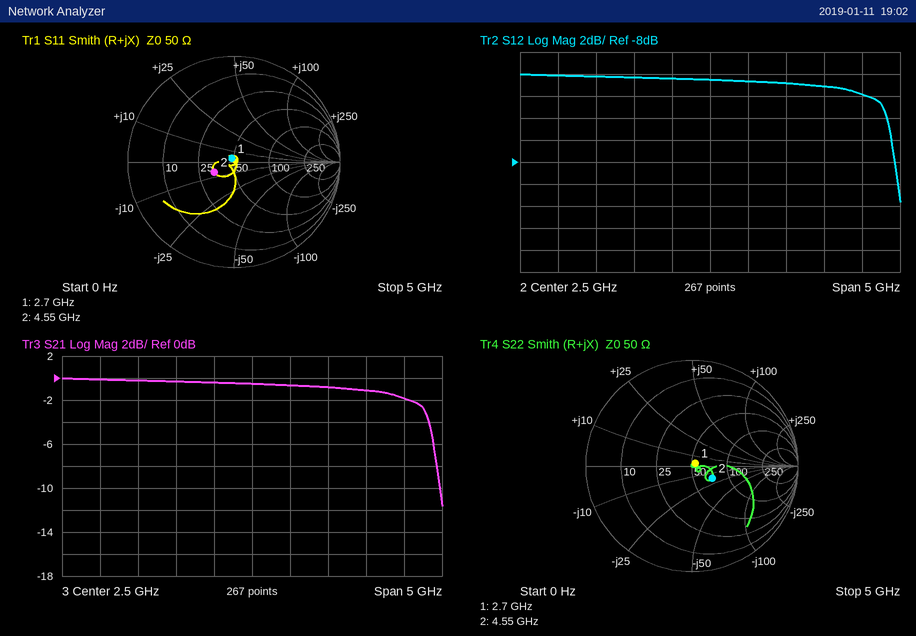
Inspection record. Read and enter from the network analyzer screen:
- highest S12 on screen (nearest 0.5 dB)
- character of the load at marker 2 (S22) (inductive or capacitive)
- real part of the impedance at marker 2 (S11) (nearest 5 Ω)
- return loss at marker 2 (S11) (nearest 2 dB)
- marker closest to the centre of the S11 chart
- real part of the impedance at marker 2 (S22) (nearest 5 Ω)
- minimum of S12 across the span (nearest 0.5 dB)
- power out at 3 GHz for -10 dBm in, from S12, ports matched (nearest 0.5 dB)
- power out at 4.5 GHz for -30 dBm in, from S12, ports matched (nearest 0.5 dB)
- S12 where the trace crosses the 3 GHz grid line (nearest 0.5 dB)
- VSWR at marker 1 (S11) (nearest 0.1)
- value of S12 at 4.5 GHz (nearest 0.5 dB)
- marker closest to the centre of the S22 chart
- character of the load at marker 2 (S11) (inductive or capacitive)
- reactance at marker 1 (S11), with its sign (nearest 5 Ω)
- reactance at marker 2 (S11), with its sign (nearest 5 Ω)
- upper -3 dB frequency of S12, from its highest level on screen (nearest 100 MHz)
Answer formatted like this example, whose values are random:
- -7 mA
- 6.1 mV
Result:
- 0.0 dB
- capacitive
- 35 Ω
- 14 dB
- marker 1
- 70 Ω
- -11.5 dB
- -10.5 dBm
- -32.0 dBm
- -0.5 dB
- 1.1
- -2.0 dB
- marker 1
- capacitive
- +5 Ω
- -5 Ω
- 4.8 GHz
